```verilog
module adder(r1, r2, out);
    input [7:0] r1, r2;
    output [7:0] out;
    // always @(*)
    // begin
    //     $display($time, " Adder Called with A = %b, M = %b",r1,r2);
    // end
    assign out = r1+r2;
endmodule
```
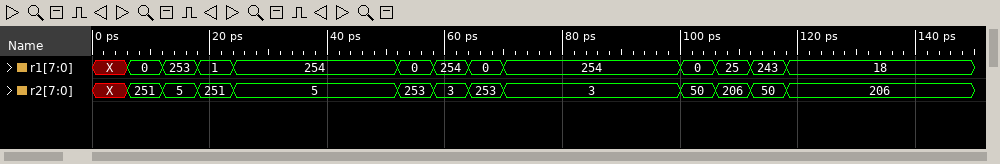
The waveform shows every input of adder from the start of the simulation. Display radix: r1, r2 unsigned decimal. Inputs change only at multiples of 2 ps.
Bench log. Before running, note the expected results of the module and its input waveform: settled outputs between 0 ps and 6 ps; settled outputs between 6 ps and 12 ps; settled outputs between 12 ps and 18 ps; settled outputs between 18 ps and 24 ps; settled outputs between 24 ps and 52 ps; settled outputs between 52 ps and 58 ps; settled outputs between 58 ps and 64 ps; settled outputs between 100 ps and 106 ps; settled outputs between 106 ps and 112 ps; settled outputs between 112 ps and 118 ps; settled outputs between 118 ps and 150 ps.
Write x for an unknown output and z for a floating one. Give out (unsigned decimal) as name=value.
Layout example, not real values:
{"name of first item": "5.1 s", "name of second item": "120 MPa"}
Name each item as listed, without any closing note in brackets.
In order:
{"settled outputs between 0 ps and 6 ps": "out=x", "settled outputs between 6 ps and 12 ps": "out=251", "settled outputs between 12 ps and 18 ps": "out=2", "settled outputs between 18 ps and 24 ps": "out=252", "settled outputs between 24 ps and 52 ps": "out=3", "settled outputs between 52 ps and 58 ps": "out=253", "settled outputs between 58 ps and 64 ps": "out=1", "settled outputs between 100 ps and 106 ps": "out=50", "settled outputs between 106 ps and 112 ps": "out=231", "settled outputs between 112 ps and 118 ps": "out=37", "settled outputs between 118 ps and 150 ps": "out=224"}
